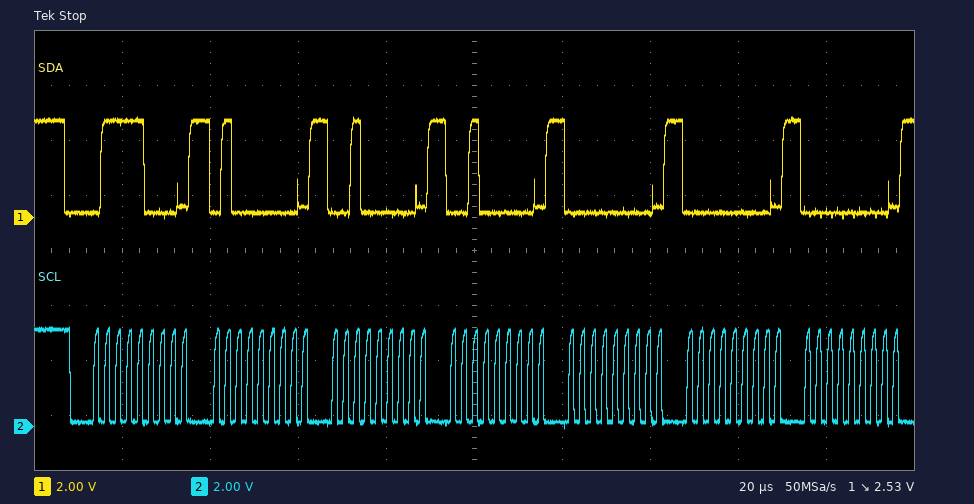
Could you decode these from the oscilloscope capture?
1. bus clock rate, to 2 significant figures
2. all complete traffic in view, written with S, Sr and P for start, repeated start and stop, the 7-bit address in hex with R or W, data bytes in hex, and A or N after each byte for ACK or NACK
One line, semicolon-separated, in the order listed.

400 kHz; S 3CW A 40 A 20 A 20 A 00 A 00 A 00 A
